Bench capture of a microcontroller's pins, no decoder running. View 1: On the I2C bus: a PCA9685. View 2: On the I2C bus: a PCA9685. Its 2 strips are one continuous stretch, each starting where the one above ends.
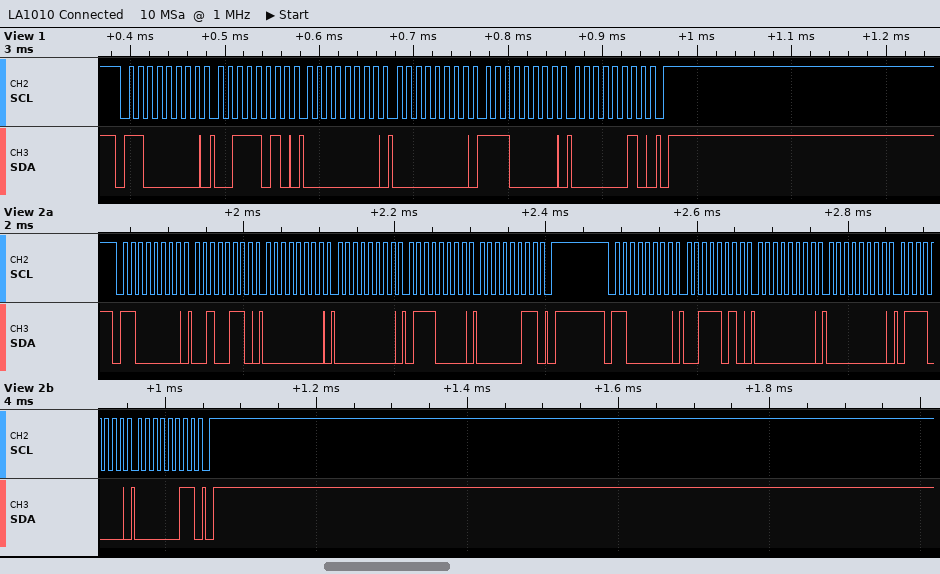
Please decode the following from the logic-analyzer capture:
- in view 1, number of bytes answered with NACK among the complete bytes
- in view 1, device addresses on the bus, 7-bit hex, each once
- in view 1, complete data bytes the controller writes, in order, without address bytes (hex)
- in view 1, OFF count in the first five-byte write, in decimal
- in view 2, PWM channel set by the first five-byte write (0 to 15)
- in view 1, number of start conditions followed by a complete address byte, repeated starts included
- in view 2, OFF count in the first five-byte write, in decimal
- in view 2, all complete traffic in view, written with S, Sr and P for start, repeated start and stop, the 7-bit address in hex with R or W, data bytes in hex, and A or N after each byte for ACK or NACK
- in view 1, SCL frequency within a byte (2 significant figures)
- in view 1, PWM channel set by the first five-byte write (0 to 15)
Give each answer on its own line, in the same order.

0
0x60
3A 00 00 E0 02
736
8
1
880
S 60W A 26 A 00 A 00 A 70 A 03 A P S 60W A 3A A 00 A 00 A 70 A 03 A P
100 kHz
13
